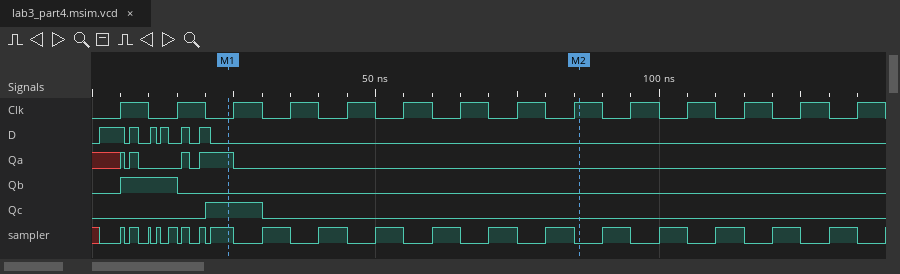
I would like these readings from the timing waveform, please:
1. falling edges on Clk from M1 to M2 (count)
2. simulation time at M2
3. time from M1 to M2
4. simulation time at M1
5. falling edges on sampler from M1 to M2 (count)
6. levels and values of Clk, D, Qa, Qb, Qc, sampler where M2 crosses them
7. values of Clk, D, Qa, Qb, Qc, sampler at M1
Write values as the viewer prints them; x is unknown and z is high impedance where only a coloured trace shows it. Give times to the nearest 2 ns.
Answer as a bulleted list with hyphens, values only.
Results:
- 6
- 86 ns
- 62 ns
- 24 ns
- 7
- Clk=1, D=0, Qa=0, Qb=0, Qc=0, sampler=0
- Clk=0, D=0, Qa=1, Qb=0, Qc=1, sampler=1
